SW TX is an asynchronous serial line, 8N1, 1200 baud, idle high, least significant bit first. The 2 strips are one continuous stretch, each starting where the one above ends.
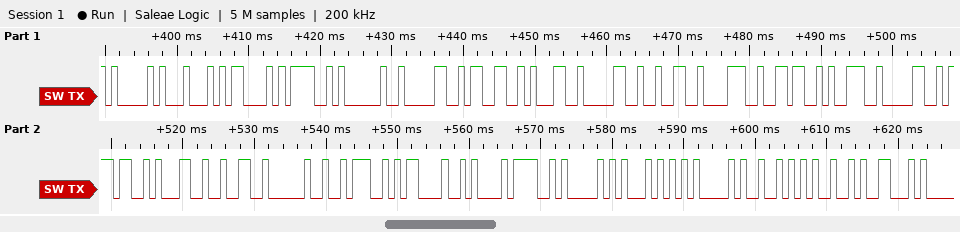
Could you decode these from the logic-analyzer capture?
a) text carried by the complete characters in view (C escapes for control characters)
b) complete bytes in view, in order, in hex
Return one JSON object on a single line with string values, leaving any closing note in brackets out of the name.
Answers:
{"text carried by the complete characters in view": "\"ADCO 031028690712 :\\r\\nOPTARIF\"", "complete bytes in view, in order, in hex": "41 44 43 4F 20 30 33 31 30 32 38 36 39 30 37 31 32 20 3A 0D 0A 4F 50 54 41 52 49 46"}
